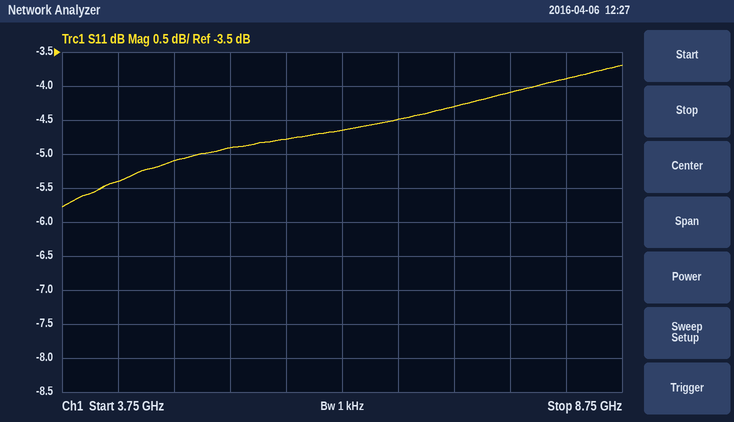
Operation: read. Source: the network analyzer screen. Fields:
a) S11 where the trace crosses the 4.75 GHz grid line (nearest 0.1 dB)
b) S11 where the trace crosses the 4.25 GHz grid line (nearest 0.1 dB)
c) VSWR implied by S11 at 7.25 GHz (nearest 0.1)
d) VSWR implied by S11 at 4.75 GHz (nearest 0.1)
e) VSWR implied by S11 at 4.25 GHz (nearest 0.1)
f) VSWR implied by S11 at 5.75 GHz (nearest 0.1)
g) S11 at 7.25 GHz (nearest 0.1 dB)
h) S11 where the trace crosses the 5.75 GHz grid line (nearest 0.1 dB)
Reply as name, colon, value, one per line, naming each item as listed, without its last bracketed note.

S11 where the trace crosses the 4.75 GHz grid line: -5.1 dB
S11 where the trace crosses the 4.25 GHz grid line: -5.4 dB
VSWR implied by S11 at 7.25 GHz: 4.1
VSWR implied by S11 at 4.75 GHz: 3.5
VSWR implied by S11 at 4.25 GHz: 3.3
VSWR implied by S11 at 5.75 GHz: 3.7
S11 at 7.25 GHz: -4.3 dB
S11 where the trace crosses the 5.75 GHz grid line: -4.8 dB
